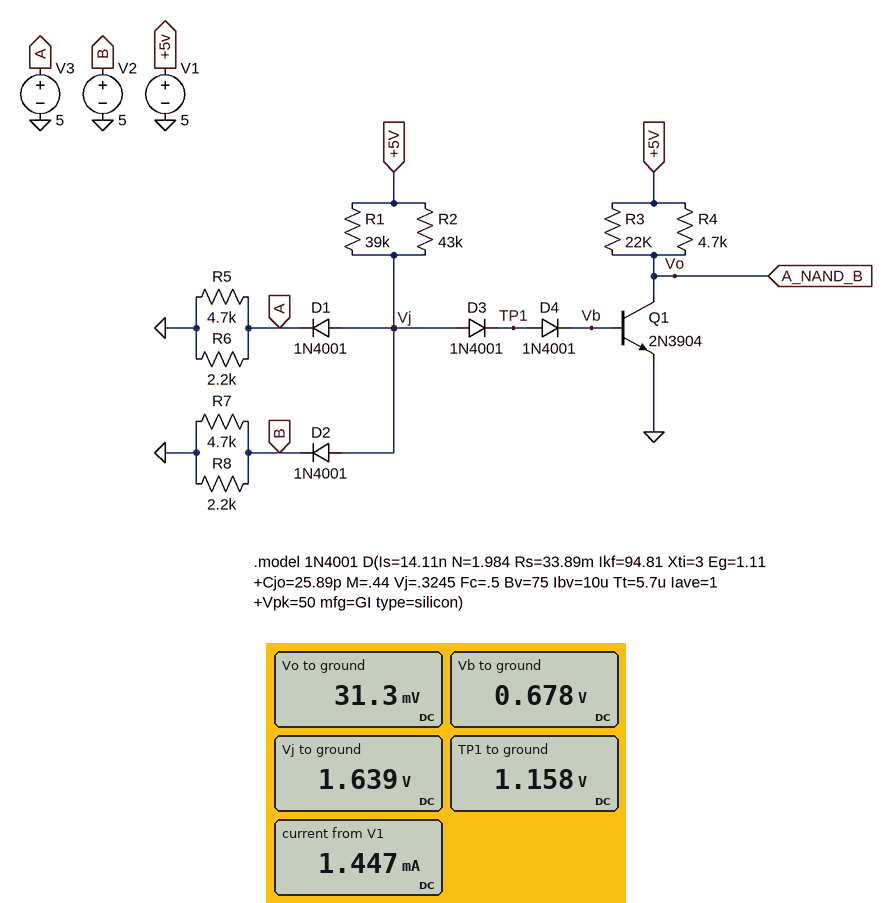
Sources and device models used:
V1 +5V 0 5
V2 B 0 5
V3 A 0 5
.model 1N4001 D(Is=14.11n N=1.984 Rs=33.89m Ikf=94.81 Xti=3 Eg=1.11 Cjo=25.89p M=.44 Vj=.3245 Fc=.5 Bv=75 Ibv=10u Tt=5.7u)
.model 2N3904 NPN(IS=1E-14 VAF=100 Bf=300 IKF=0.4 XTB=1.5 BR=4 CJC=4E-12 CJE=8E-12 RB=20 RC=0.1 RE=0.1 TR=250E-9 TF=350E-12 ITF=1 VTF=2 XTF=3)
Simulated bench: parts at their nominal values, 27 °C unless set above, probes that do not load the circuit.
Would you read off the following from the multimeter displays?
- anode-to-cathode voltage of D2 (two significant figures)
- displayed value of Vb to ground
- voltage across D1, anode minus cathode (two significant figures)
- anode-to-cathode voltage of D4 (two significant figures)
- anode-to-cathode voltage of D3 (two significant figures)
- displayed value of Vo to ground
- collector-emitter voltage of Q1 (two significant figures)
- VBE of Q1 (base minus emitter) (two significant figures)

-3.4 V
0.678 V
-3.4 V
480 mV
480 mV
31.3 mV
31 mV
680 mV
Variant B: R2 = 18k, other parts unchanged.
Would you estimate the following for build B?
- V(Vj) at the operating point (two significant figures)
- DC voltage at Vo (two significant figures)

1.7 V
24 mV
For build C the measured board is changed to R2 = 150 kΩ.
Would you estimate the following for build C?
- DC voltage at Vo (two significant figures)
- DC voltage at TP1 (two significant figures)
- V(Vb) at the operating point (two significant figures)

38 mV
1.1 V
670 mV
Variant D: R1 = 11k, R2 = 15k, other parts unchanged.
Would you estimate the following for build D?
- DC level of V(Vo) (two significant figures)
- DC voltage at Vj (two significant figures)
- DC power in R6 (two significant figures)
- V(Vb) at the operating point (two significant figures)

17 mV
1.8 V
11 mW
700 mV
